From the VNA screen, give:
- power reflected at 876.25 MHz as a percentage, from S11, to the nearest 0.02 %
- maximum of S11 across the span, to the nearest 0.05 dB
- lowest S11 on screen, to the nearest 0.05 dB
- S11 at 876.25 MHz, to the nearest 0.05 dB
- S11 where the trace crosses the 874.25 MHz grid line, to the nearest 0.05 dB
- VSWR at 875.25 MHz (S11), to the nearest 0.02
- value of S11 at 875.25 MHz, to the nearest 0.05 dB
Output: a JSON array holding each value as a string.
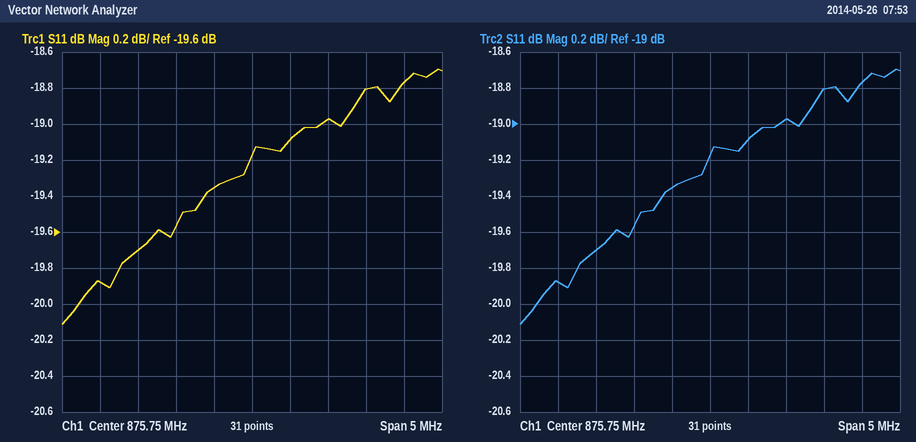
["1.24 %", "-18.70 dB", "-20.10 dB", "-19.10 dB", "-19.70 dB", "1.24", "-19.35 dB"]
